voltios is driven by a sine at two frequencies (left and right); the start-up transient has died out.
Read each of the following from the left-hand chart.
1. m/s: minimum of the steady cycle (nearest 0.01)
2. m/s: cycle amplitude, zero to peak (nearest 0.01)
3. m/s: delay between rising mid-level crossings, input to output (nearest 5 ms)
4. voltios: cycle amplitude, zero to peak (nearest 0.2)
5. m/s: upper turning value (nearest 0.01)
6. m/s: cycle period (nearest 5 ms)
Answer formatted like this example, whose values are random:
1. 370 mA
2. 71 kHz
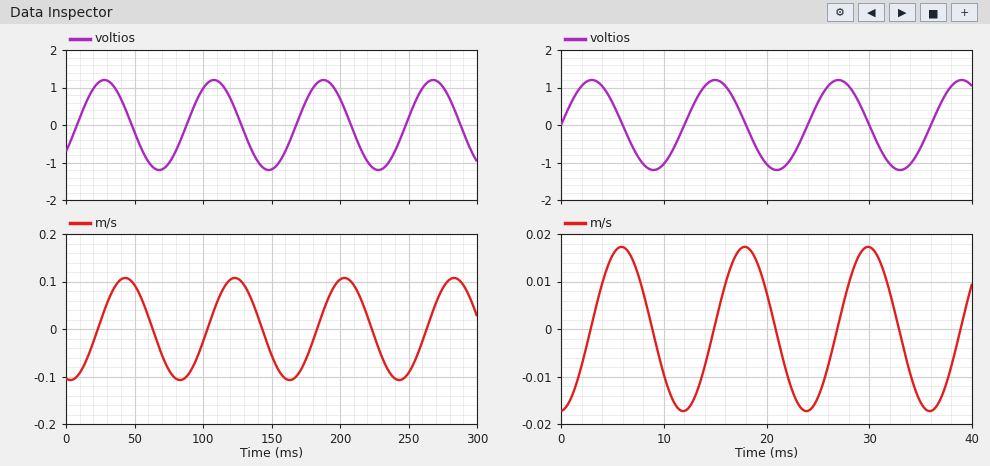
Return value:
1. -0.11
2. 0.11
3. 15 ms
4. 1.2
5. 0.11
6. 80 ms
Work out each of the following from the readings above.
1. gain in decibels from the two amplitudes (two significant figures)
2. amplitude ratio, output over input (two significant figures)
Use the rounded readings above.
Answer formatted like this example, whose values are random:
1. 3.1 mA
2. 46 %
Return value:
1. -21 dB
2. 0.092
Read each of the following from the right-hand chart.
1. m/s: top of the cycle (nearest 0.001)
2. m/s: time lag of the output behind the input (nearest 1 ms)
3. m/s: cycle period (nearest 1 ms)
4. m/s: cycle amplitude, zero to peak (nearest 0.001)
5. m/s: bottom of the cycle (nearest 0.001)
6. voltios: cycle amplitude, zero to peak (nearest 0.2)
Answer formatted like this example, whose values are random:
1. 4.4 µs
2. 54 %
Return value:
1. 0.017
2. 3 ms
3. 12 ms
4. 0.017
5. -0.017
6. 1.2
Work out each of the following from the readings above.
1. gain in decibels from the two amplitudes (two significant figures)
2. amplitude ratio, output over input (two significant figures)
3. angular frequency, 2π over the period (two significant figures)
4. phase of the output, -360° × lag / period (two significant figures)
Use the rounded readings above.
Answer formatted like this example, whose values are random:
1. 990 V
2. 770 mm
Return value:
1. -37 dB
2. 0.014
3. 0.52 rad/ms
4. -90°
